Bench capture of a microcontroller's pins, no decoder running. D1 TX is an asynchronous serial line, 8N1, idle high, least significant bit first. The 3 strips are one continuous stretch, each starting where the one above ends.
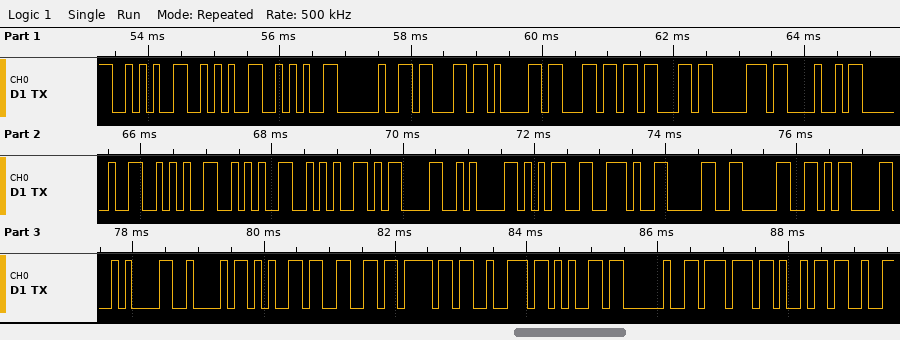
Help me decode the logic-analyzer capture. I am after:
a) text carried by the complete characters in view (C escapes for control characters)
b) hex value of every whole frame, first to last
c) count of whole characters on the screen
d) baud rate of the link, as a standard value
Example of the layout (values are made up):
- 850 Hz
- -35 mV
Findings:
- "*** calcpH ***\r\n5.00\r\nBefore wi"
- 0x2A 0x2A 0x2A 0x20 0x63 0x61 0x6C 0x63 0x70 0x48 0x20 0x2A 0x2A 0x2A 0x0D 0x0A 0x35 0x2E 0x30 0x30 0x0D 0x0A 0x42 0x65 0x66 0x6F 0x72 0x65 0x20 0x77 0x69
- 31
- 9600 baud
